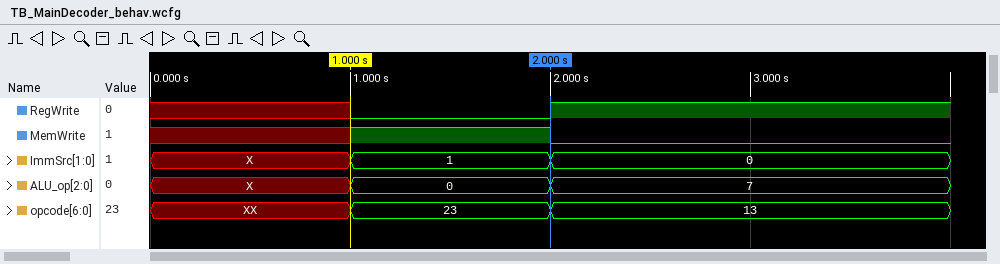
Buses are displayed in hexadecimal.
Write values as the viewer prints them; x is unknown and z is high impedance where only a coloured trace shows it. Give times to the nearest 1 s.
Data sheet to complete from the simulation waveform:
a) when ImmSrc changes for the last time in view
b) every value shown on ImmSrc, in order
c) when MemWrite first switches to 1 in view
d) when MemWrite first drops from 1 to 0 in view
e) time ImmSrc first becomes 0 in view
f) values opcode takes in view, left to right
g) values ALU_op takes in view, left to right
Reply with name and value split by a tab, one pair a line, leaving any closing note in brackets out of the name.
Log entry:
when ImmSrc changes for the last time in view	2 s
every value shown on ImmSrc, in order	X, 1, 0
when MemWrite first switches to 1 in view	1 s
when MemWrite first drops from 1 to 0 in view	2 s
time ImmSrc first becomes 0 in view	2 s
values opcode takes in view, left to right	XX, 23, 13
values ALU_op takes in view, left to right	X, 0, 7
